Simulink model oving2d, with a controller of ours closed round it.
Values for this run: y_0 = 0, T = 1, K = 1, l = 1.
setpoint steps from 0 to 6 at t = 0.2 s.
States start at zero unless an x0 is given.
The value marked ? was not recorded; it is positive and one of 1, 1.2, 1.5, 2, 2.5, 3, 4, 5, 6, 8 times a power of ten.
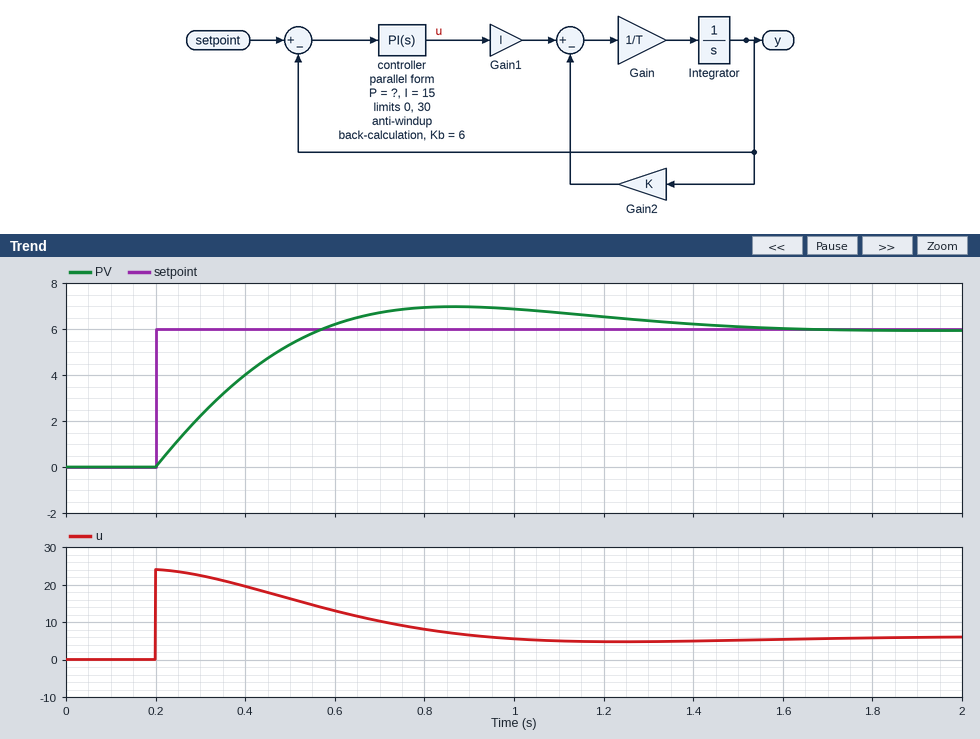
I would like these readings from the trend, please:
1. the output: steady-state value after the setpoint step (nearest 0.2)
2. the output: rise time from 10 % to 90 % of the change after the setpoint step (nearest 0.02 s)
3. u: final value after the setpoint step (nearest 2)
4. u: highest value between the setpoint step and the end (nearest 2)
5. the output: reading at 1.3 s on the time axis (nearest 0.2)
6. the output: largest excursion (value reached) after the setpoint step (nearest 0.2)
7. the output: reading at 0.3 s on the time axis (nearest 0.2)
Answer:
6.0
0.28 s
6
24
6.4
7.0
2.2
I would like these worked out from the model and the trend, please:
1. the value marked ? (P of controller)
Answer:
4
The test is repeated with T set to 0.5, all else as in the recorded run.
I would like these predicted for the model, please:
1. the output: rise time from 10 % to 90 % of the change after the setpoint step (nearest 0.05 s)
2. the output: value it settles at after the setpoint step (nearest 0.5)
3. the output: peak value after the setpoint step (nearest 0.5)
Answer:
0.20 s
6.0
6.5
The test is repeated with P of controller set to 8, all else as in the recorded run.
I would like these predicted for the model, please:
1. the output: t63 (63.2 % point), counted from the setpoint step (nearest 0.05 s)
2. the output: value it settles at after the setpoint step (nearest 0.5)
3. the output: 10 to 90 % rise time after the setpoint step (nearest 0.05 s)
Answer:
0.15 s
6.0
0.25 s
